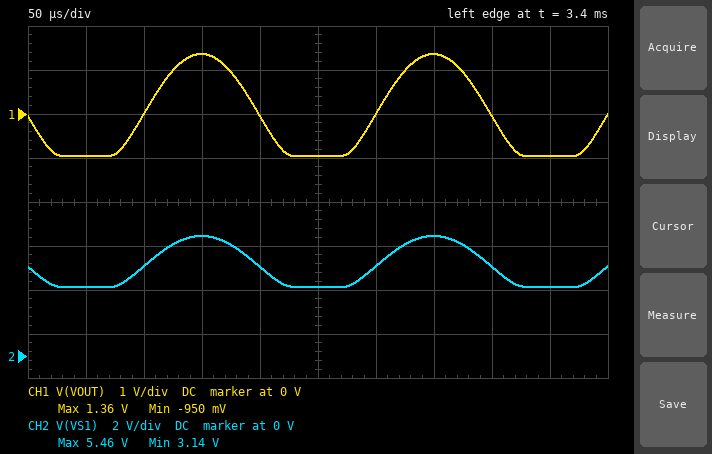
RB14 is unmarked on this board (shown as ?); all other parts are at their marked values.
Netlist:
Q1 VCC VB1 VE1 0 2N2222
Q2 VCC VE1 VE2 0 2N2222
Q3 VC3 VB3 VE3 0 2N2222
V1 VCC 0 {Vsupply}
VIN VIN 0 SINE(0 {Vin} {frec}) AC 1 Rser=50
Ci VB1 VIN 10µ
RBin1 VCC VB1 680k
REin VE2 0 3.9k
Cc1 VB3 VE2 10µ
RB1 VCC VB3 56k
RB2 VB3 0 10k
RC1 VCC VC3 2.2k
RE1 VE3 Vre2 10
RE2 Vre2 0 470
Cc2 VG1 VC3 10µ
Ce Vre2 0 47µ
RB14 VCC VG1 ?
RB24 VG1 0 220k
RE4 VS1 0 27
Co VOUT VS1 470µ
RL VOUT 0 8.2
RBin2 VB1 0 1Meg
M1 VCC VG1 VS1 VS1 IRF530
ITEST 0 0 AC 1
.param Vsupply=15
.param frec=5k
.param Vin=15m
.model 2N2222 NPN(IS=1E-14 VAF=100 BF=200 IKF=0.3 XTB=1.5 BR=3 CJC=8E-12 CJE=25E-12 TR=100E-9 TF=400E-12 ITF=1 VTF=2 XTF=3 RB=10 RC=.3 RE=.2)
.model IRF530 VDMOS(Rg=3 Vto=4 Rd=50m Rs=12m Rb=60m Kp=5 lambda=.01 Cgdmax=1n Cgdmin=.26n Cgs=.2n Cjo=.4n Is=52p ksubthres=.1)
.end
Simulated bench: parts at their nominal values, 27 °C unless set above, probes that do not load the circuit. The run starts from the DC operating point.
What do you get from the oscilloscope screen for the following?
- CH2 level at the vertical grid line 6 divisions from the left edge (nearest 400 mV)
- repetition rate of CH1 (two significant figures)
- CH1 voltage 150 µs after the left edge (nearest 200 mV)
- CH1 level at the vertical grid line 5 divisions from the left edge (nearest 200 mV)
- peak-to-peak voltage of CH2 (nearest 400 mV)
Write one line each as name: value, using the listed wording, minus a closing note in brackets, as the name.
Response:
CH2 level at the vertical grid line 6 divisions from the left edge: 4.0 V
repetition rate of CH1: 5.0 kHz
CH1 voltage 150 µs after the left edge: 1.4 V
CH1 level at the vertical grid line 5 divisions from the left edge: -1.0 V
peak-to-peak voltage of CH2: 2.4 V
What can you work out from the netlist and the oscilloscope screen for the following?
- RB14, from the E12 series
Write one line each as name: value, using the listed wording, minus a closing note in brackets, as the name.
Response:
RB14, from the E12 series: 180 kΩ
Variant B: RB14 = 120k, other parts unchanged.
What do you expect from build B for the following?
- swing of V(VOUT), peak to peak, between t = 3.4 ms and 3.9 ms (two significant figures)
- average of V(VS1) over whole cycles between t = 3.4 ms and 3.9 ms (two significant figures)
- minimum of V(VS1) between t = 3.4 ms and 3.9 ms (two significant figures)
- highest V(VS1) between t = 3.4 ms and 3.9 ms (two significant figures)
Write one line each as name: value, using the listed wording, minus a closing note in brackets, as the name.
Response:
swing of V(VOUT), peak to peak, between t = 3.4 ms and 3.9 ms: 2.7 V
average of V(VS1) over whole cycles between t = 3.4 ms and 3.9 ms: 5.5 V
minimum of V(VS1) between t = 3.4 ms and 3.9 ms: 4.2 V
highest V(VS1) between t = 3.4 ms and 3.9 ms: 6.9 V
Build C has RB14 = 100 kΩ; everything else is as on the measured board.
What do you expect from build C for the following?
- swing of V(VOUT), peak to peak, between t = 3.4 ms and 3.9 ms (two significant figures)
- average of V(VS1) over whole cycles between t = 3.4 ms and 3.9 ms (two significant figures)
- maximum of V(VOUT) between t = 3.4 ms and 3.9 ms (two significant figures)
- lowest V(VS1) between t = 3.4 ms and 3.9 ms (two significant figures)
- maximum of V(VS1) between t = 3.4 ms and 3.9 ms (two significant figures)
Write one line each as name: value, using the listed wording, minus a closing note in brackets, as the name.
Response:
swing of V(VOUT), peak to peak, between t = 3.4 ms and 3.9 ms: 2.8 V
average of V(VS1) over whole cycles between t = 3.4 ms and 3.9 ms: 6.1 V
maximum of V(VOUT) between t = 3.4 ms and 3.9 ms: 1.4 V
lowest V(VS1) between t = 3.4 ms and 3.9 ms: 4.7 V
maximum of V(VS1) between t = 3.4 ms and 3.9 ms: 7.5 V
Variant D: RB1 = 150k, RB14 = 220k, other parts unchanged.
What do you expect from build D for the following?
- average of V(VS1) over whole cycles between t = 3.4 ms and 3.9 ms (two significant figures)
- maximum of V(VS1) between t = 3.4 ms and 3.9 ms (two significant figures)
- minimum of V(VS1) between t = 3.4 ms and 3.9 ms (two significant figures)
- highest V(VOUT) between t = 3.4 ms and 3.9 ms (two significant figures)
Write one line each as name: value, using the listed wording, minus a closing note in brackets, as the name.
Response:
average of V(VS1) over whole cycles between t = 3.4 ms and 3.9 ms: 3.3 V
maximum of V(VS1) between t = 3.4 ms and 3.9 ms: 3.7 V
minimum of V(VS1) between t = 3.4 ms and 3.9 ms: 2.8 V
highest V(VOUT) between t = 3.4 ms and 3.9 ms: 450 mV
